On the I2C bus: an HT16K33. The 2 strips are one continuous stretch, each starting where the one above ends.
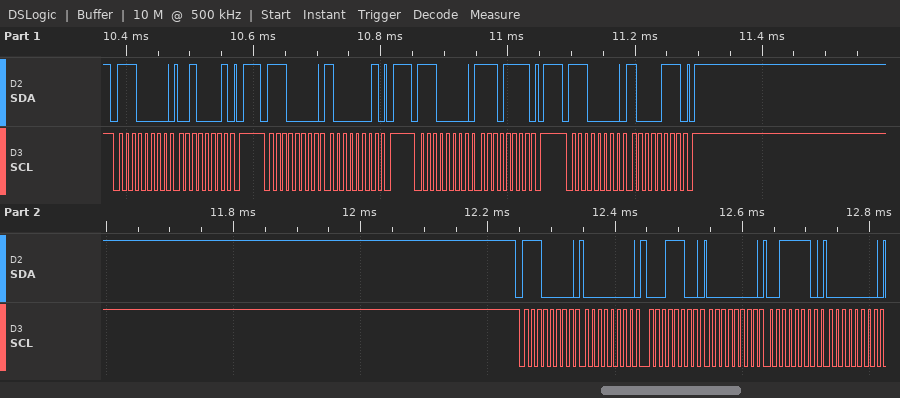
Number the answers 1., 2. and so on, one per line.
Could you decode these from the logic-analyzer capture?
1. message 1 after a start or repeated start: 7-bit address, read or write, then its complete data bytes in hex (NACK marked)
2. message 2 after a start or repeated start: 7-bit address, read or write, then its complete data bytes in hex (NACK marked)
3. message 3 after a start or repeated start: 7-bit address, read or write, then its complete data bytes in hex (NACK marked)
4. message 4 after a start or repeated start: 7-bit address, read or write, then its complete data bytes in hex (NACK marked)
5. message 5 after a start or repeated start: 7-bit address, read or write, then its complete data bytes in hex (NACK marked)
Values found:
1. 0x70 write: 21
2. 0x70 write: 81
3. 0x70 write: EF
4. 0x70 write: 87
5. 0x70 write: 00 1C 00 3E 00
